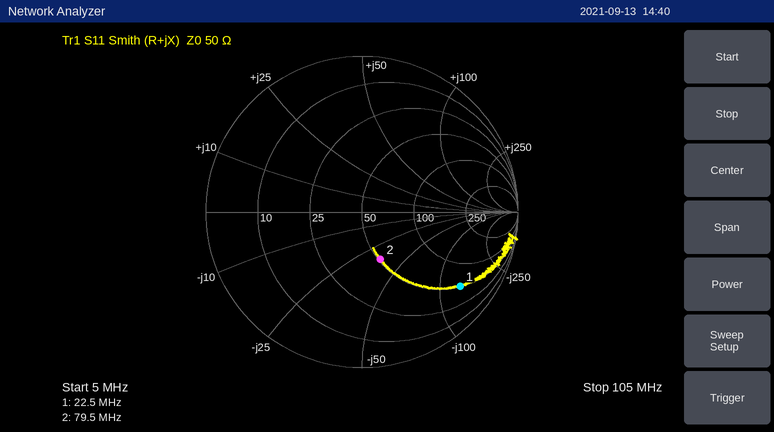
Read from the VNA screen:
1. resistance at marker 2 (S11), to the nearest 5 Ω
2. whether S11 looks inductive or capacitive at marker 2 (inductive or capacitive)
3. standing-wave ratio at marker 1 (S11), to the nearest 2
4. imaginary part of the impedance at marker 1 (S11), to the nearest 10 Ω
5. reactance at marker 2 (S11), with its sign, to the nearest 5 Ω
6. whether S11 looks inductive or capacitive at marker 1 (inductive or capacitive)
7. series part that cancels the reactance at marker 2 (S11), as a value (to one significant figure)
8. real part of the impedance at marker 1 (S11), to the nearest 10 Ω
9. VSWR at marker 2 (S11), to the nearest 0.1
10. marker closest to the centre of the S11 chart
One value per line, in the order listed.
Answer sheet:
50 Ω
capacitive
8
-130 Ω
-35 Ω
capacitive
70 nH
50 Ω
2.0
marker 2
